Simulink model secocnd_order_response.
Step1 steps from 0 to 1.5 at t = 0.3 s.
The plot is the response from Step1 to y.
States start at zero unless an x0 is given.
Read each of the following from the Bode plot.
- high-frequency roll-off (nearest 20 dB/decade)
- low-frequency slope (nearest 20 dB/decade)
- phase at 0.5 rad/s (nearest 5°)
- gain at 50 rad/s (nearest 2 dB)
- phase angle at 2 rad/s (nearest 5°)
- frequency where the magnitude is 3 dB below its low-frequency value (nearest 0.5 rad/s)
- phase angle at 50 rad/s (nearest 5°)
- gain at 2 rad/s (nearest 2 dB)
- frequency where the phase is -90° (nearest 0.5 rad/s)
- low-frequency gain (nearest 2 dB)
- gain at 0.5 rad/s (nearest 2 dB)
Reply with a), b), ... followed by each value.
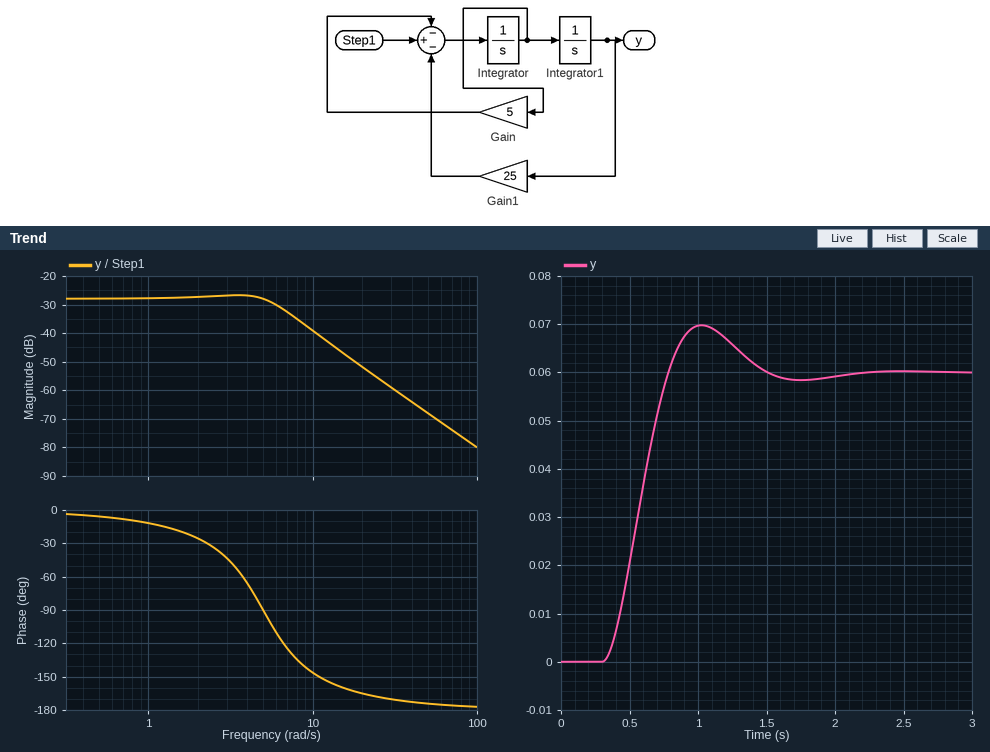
a) -40 dB/decade
b) 0 dB/decade
c) -5°
d) -68 dB
e) -25°
f) 6.5 rad/s
g) -175°
h) -28 dB
i) 5.0 rad/s
j) -28 dB
k) -28 dB
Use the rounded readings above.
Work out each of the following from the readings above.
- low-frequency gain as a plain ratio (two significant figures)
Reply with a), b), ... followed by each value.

a) 0.040
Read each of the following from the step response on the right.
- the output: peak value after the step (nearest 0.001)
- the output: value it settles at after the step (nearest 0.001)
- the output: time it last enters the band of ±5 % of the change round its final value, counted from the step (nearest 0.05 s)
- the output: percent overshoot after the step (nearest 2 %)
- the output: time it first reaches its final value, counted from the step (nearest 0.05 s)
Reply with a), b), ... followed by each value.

a) 0.070
b) 0.060
c) 1.05 s
d) 16 %
e) 0.50 s
